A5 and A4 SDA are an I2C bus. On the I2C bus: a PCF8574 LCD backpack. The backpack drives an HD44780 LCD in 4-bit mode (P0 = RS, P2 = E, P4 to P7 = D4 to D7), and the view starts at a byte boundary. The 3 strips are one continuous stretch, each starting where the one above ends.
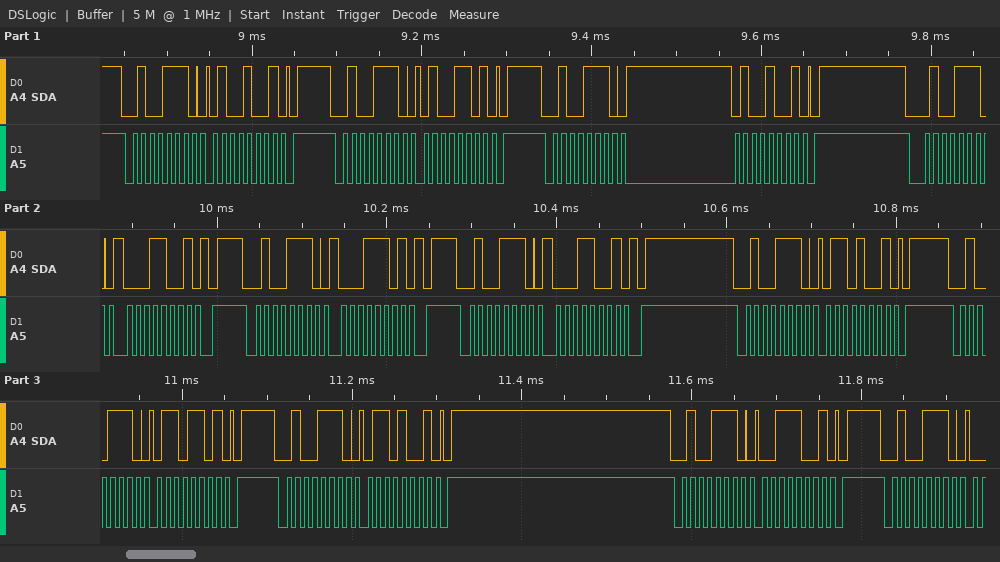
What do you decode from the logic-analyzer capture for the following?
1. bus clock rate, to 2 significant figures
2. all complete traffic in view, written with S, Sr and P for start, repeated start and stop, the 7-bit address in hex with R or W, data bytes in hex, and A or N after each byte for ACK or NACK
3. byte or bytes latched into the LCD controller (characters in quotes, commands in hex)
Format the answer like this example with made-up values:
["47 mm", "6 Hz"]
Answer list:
["100 kHz", "S 27W A 49 A P S 27W A 4D A P S 27W A 49 A P S 27W A 19 A P S 27W A 1D A P S 27W A 19 A P S 27W A 69 A P S 27W A 6D A P S 27W A 69 A P S 27W A 39 A P S 27W A", "'A'"]
